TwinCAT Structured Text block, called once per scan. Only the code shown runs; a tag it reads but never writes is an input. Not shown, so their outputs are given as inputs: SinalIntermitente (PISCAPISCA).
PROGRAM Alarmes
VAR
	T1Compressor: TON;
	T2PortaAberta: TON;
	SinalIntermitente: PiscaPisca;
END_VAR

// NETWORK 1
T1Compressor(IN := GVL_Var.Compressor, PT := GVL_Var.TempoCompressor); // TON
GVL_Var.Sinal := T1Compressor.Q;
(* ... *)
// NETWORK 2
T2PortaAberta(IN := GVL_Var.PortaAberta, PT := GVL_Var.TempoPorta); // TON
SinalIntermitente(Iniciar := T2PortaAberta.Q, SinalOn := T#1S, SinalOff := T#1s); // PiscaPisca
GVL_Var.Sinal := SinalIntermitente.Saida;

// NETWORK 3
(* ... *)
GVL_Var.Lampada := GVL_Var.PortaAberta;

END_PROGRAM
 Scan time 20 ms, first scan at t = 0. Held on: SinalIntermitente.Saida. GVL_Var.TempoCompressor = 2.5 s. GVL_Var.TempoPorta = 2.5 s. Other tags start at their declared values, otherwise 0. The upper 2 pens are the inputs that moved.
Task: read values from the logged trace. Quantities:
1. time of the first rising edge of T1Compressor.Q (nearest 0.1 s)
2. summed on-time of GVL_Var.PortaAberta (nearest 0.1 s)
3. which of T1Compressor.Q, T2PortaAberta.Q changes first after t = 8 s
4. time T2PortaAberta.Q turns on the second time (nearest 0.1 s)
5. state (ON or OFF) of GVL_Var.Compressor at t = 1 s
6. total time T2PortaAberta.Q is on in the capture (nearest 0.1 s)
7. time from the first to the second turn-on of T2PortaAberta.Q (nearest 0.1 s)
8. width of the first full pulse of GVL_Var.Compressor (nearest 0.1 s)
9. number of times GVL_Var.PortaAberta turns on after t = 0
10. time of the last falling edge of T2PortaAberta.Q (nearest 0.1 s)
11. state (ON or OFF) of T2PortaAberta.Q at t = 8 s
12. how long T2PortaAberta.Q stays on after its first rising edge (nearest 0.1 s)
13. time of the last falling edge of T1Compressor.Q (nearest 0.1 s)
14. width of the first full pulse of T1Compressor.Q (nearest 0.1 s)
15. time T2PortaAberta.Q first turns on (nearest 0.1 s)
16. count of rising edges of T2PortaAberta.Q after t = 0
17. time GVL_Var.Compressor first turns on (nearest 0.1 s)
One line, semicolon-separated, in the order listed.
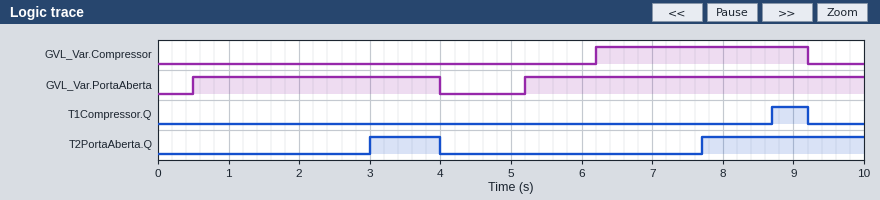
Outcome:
8.7 s; 8.3 s; T1Compressor.Q; 7.7 s; OFF; 3.3 s; 4.7 s; 3.0 s; 2; 4.0 s; ON; 1.0 s; 9.2 s; 0.5 s; 3.0 s; 2; 6.2 s
